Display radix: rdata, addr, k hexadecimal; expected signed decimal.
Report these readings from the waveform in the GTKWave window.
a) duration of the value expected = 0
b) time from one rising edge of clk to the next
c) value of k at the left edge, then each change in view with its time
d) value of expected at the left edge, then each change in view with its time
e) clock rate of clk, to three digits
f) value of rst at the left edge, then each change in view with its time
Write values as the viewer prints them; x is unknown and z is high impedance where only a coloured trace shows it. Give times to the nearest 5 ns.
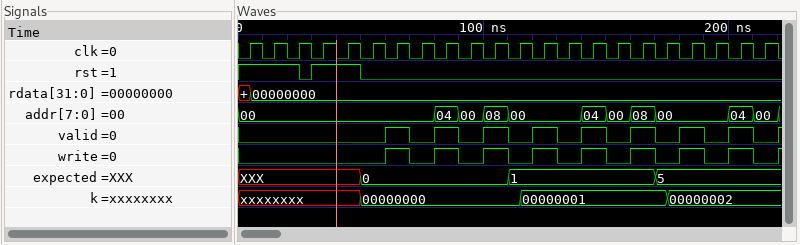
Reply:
60 ns
10 ns
xxxxxxxx, 00000000 at 50 ns, 00000001 at 115 ns, 00000002 at 175 ns
XXX, 0 at 50 ns, 1 at 110 ns, 5 at 170 ns
100 MHz
1, 0 at 25 ns, 1 at 30 ns, 0 at 50 ns
